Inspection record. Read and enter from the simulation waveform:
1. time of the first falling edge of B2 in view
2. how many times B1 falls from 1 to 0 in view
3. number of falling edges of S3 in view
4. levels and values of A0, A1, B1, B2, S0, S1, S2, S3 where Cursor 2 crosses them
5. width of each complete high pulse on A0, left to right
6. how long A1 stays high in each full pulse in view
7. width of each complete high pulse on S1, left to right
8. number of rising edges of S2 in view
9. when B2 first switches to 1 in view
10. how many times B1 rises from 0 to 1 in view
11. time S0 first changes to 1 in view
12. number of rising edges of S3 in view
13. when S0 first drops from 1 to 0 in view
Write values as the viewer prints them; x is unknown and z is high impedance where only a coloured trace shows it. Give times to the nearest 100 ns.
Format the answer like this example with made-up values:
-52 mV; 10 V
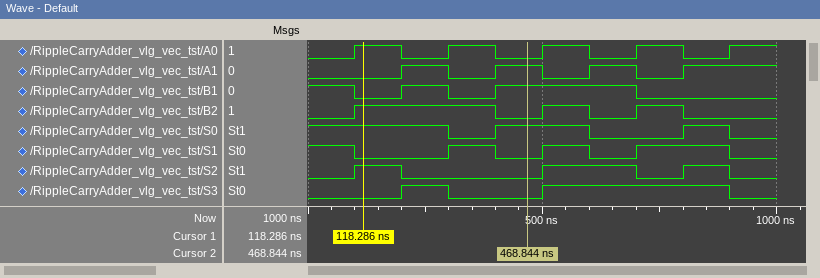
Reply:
400 ns; 3; 2; A0=0, A1=1, B1=1, B2=0, S0=1, S1=0, S2=0, S3=0; 100 ns, 100 ns, 100 ns, 100 ns; 100 ns, 100 ns, 100 ns; 100 ns, 100 ns, 200 ns; 3; 100 ns; 2; 400 ns; 2; 300 ns
